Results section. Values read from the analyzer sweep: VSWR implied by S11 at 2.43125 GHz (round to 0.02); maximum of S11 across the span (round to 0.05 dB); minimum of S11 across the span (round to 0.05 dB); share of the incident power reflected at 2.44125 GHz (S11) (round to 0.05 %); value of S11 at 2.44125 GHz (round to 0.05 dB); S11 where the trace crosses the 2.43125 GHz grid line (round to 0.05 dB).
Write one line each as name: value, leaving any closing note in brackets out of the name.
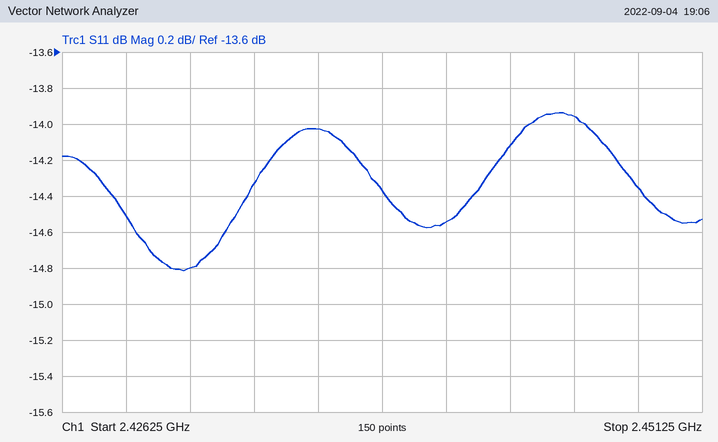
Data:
VSWR implied by S11 at 2.43125 GHz: 1.44
maximum of S11 across the span: -13.95 dB
minimum of S11 across the span: -14.80 dB
share of the incident power reflected at 2.44125 GHz (S11): 3.50 %
value of S11 at 2.44125 GHz: -14.55 dB
S11 where the trace crosses the 2.43125 GHz grid line: -14.80 dB
